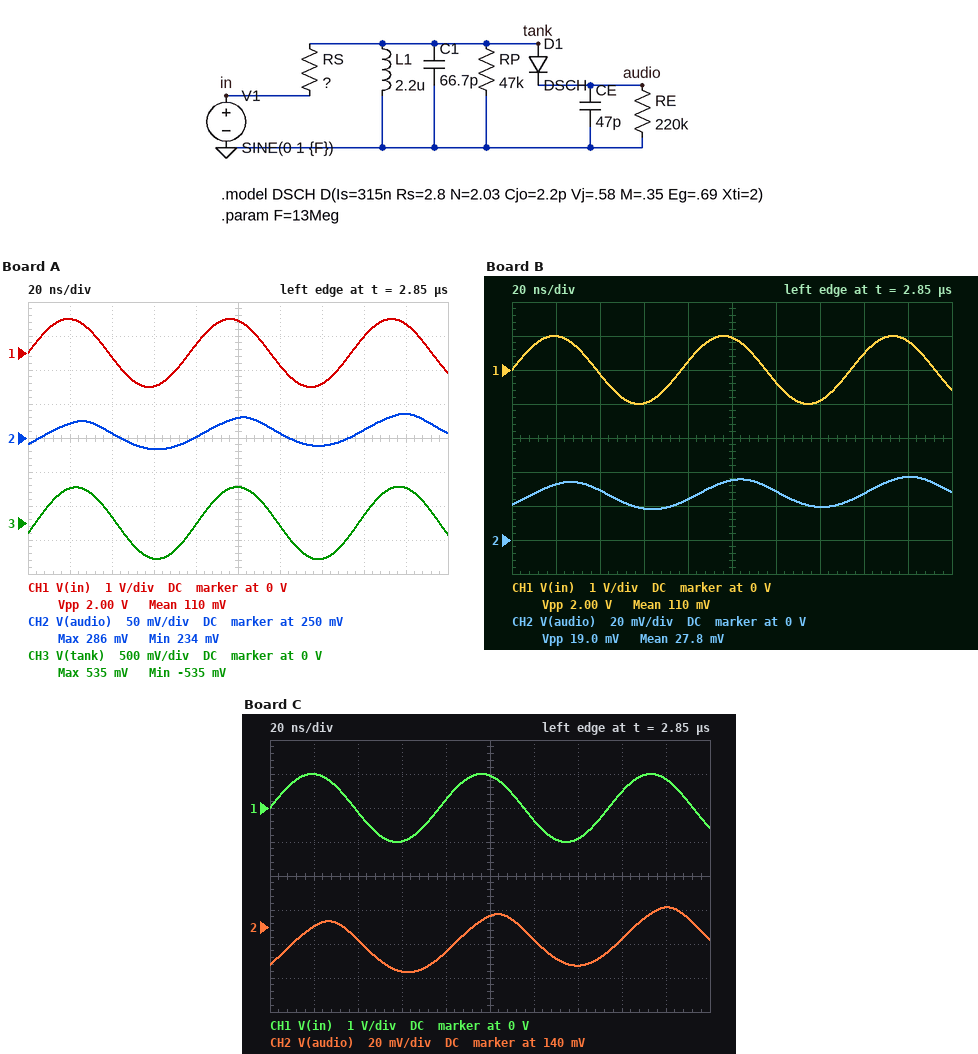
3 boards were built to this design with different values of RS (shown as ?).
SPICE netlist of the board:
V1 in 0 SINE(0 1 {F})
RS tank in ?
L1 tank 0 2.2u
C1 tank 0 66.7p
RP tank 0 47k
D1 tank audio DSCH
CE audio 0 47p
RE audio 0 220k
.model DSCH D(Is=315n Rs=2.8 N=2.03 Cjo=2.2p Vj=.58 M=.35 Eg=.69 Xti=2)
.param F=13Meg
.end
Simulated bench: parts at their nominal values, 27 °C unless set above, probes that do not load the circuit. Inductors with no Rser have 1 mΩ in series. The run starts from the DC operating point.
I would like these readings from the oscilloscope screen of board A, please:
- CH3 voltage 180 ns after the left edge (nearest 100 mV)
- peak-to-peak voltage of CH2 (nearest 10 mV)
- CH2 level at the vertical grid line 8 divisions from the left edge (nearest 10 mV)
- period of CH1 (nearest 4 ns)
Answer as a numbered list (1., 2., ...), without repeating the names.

1. 500 mV
2. 50 mV
3. 260 mV
4. 76 ns
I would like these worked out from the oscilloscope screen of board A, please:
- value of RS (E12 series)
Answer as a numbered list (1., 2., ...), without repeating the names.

1. 15 kΩ
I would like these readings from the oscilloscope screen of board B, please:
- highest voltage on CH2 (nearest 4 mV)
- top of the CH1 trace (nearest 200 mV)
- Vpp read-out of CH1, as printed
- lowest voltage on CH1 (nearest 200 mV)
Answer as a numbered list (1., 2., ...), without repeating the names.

1. 36 mV
2. 1.0 V
3. 2.00 V
4. -1.0 V
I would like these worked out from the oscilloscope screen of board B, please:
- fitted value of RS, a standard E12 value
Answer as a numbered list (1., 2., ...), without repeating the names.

1. 68 kΩ
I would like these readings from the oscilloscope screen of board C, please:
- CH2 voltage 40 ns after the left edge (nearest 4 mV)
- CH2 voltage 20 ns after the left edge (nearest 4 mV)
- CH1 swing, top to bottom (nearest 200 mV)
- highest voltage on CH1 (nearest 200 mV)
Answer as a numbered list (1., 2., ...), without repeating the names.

1. 132 mV
2. 140 mV
3. 2.0 V
4. 1.0 V
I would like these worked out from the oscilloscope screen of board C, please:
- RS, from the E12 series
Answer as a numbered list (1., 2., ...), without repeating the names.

1. 27 kΩ
